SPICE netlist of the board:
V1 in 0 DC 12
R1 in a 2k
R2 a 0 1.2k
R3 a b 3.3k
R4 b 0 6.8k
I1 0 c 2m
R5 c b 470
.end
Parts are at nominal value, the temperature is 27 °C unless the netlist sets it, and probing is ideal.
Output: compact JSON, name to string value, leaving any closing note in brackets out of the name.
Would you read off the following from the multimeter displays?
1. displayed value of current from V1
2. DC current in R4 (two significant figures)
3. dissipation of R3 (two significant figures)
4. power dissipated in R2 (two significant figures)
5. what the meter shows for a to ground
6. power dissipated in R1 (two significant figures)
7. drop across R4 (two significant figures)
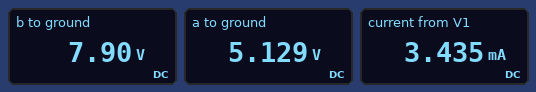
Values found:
{"displayed value of current from V1": "3.435 mA", "DC current in R4": "1.2 mA", "dissipation of R3": "2.3 mW", "power dissipated in R2": "22 mW", "what the meter shows for a to ground": "5.129 V", "power dissipated in R1": "24 mW", "drop across R4": "7.9 V"}
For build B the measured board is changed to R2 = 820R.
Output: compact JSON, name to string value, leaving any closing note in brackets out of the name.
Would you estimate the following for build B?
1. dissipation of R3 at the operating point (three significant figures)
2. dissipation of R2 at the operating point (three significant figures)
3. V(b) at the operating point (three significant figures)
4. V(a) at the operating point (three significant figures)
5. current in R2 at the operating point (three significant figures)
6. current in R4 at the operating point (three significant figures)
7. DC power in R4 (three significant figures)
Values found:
{"dissipation of R3 at the operating point": "2.96 mW", "dissipation of R2 at the operating point": "19.9 mW", "V(b) at the operating point": "7.16 V", "V(a) at the operating point": "4.04 V", "current in R2 at the operating point": "4.93 mA", "current in R4 at the operating point": "1.05 mA", "DC power in R4": "7.55 mW"}
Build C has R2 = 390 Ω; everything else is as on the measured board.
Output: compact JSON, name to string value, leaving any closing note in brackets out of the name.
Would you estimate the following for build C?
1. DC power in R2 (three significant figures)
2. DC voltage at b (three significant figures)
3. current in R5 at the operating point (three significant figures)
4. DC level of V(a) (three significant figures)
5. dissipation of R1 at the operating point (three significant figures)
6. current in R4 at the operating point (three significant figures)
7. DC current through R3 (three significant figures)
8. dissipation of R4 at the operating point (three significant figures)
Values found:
{"DC power in R2": "13.8 mW", "DC voltage at b": "6.01 V", "current in R5 at the operating point": "2.00 mA", "DC level of V(a)": "2.32 V", "dissipation of R1 at the operating point": "46.8 mW", "current in R4 at the operating point": "883 µA", "DC current through R3": "1.12 mA", "dissipation of R4 at the operating point": "5.31 mW"}
